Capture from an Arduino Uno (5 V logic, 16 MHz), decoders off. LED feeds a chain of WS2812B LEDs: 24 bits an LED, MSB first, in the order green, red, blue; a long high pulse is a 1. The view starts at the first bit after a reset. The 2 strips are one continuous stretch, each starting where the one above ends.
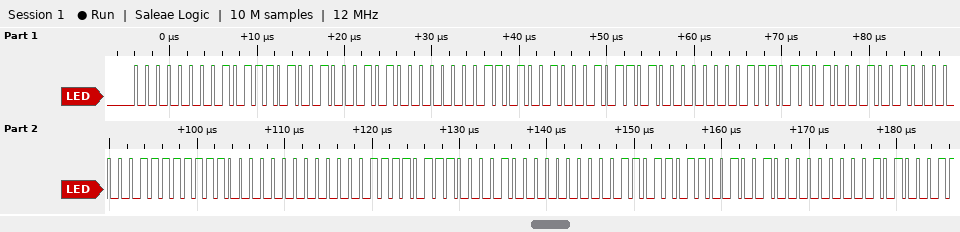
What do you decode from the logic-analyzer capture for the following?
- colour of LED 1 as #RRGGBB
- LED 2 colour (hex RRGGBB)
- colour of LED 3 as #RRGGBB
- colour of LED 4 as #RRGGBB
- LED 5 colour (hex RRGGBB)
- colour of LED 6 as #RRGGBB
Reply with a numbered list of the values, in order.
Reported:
1. #BA0045
2. #D2002D
3. #ED0012
4. #FC0300
5. #E11E00
6. #C93600
